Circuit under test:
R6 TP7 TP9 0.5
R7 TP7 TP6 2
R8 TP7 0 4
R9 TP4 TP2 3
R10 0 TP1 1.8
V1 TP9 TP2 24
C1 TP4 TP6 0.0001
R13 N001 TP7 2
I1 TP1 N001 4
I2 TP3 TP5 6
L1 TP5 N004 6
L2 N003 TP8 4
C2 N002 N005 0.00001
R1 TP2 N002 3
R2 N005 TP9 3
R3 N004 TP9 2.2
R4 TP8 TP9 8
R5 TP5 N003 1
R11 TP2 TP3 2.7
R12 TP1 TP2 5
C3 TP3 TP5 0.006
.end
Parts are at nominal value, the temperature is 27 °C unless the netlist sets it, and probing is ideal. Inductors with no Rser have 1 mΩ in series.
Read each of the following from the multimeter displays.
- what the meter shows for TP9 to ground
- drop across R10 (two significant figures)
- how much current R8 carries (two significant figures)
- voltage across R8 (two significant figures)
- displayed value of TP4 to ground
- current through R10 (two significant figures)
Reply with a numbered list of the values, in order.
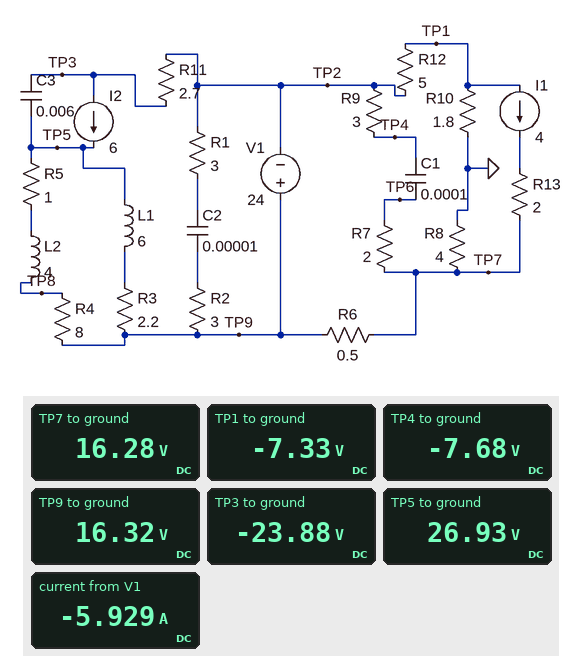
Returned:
1. 16.32 V
2. 7.3 V
3. 4.1 A
4. 16 V
5. -7.68 V
6. 4.1 A
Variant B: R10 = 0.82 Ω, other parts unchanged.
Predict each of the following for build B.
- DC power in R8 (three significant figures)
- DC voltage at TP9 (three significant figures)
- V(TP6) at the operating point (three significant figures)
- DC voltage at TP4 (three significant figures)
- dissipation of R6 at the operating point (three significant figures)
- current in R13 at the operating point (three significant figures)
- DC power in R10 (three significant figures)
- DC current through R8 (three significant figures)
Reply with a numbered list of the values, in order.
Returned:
1. 79.5 W
2. 18.1 V
3. 17.8 V
4. -5.94 V
5. 105 mW
6. 4.00 A
7. 16.3 W
8. 4.46 A
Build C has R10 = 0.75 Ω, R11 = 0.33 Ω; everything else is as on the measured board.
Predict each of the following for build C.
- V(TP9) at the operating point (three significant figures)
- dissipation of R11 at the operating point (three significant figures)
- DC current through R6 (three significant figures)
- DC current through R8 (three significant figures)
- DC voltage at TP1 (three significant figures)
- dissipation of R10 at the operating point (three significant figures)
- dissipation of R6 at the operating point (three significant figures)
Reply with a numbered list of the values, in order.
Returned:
1. 18.2 V
2. 11.9 W
3. 488 mA
4. 4.49 A
5. -3.37 V
6. 15.1 W
7. 119 mW
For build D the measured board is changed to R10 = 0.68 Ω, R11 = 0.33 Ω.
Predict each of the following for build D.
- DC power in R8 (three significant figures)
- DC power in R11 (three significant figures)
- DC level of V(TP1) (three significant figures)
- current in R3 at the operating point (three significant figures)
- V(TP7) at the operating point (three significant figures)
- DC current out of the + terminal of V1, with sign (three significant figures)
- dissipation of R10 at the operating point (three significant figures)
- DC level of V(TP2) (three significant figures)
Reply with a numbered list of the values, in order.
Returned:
1. 81.7 W
2. 11.9 W
3. -3.07 V
4. 4.82 A
5. 18.1 V
6. -5.48 A
7. 13.9 W
8. -5.67 V
